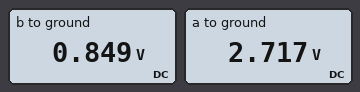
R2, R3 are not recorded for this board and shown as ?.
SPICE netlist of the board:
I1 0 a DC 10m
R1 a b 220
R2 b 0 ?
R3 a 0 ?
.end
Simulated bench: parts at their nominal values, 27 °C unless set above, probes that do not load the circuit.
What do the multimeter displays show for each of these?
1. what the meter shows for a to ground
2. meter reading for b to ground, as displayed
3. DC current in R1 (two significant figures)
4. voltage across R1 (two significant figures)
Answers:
2.717 V
0.849 V
8.5 mA
1.9 V
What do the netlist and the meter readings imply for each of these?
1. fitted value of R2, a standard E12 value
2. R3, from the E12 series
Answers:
100 Ω
1.8 kΩ
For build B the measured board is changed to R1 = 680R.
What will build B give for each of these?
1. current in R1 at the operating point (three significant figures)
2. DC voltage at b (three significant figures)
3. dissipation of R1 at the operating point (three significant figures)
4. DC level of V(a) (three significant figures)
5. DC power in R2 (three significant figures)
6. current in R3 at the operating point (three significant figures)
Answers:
6.98 mA
698 mV
33.1 mW
5.44 V
4.87 mW
3.02 mA
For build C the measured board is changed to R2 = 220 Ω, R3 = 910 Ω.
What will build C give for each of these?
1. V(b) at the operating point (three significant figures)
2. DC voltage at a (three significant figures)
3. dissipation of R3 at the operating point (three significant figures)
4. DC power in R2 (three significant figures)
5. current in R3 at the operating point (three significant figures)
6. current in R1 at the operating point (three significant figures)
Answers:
1.48 V
2.97 V
9.67 mW
10.0 mW
3.26 mA
6.74 mA
